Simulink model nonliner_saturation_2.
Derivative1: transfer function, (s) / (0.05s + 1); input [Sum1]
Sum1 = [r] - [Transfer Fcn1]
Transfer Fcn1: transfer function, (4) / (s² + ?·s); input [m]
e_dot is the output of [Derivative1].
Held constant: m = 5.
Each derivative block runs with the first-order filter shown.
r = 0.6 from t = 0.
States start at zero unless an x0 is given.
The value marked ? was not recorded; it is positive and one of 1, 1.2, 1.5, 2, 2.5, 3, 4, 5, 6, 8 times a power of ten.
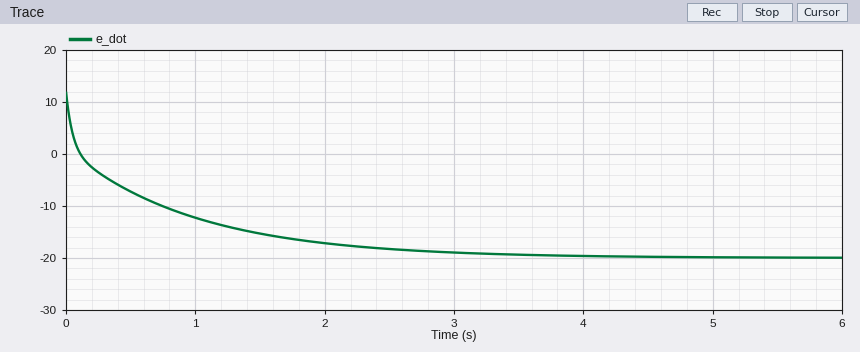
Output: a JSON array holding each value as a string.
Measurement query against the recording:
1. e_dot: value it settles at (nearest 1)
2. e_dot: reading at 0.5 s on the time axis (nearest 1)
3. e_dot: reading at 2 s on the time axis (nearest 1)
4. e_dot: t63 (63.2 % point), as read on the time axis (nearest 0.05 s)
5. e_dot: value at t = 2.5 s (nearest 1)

["-20", "-7", "-17", "0.60 s", "-18"]
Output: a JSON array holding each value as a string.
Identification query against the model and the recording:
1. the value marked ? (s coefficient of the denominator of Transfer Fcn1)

["1"]
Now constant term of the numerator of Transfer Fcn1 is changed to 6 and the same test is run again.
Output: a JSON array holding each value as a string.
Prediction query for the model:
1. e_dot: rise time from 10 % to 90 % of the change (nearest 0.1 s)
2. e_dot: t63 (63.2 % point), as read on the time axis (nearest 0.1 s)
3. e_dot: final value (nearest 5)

["2.0 s", "0.7 s", "-30"]
